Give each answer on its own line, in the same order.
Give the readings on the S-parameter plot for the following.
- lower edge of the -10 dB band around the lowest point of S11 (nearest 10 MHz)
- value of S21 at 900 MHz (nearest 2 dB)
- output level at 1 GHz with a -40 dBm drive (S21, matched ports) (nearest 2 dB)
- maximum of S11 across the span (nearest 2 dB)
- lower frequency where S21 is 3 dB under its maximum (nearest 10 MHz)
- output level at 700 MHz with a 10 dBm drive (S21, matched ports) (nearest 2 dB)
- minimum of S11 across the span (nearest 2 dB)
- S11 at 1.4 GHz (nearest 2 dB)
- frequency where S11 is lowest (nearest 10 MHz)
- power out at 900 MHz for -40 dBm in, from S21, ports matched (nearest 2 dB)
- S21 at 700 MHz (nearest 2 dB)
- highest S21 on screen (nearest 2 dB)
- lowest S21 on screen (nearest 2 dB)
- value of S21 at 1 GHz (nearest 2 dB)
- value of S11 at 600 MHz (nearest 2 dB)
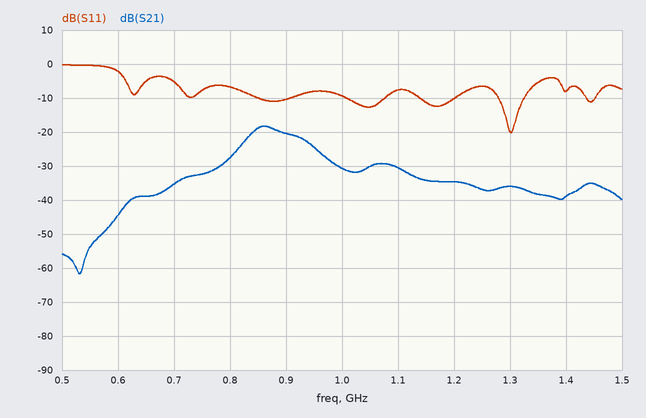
1.28 GHz
-20 dB
-70 dBm
0 dB
830 MHz
-26 dBm
-20 dB
-8 dB
1.30 GHz
-60 dBm
-36 dB
-18 dB
-62 dB
-30 dB
-2 dB
